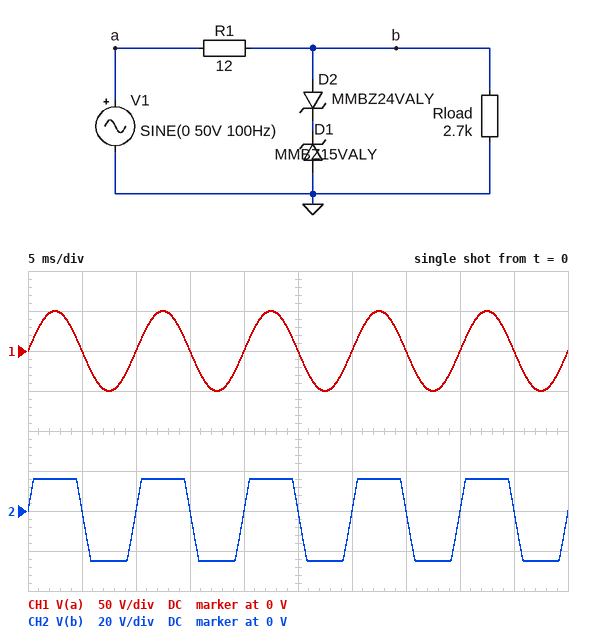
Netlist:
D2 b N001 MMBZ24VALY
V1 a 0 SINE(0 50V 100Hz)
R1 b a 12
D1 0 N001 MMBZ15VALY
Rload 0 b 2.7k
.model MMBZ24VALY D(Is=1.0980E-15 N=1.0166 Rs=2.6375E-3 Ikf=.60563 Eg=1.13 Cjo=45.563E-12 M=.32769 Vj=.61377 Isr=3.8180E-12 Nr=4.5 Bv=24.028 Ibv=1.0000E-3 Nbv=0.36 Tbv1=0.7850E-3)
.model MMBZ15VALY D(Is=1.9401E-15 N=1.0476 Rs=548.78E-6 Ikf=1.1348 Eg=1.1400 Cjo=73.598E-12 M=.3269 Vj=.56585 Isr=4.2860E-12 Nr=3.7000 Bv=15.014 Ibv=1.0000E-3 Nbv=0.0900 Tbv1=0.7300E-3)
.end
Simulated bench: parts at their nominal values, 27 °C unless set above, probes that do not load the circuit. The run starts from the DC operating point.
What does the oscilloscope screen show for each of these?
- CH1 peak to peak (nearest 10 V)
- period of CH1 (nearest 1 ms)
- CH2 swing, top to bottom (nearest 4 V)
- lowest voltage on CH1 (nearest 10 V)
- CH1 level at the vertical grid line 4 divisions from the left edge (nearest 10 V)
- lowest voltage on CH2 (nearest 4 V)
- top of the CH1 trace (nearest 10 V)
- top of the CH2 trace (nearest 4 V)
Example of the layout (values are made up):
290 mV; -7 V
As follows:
100 V; 10 ms; 40 V; -50 V; 0 V; -24 V; 50 V; 16 V
